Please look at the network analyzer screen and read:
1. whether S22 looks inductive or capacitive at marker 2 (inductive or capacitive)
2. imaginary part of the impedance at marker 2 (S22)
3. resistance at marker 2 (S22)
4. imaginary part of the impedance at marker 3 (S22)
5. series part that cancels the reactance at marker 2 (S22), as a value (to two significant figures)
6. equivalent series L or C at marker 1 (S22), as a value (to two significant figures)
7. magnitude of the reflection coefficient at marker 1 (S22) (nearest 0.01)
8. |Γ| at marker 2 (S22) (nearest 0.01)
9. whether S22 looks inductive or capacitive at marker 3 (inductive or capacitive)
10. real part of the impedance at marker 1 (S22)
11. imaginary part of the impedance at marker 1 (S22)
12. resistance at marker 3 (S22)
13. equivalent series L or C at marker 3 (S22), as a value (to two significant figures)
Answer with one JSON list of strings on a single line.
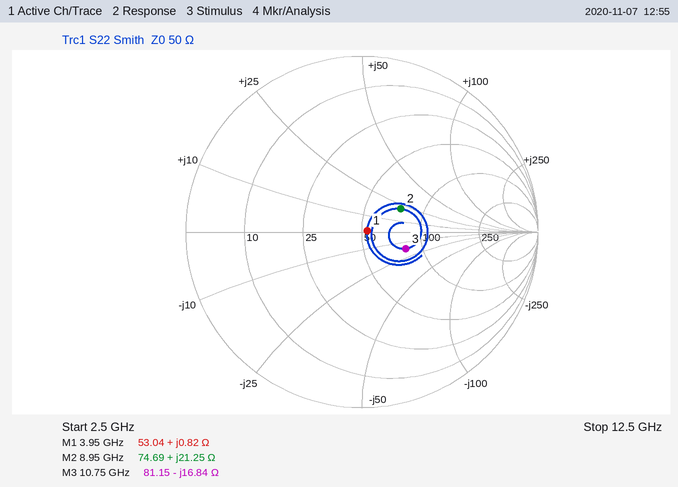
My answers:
["inductive", "+21.25 Ω", "74.69 Ω", "-16.84 Ω", "840 fF", "33 pH", "0.03", "0.26", "capacitive", "53.04 Ω", "+0.82 Ω", "81.15 Ω", "880 fF"]
